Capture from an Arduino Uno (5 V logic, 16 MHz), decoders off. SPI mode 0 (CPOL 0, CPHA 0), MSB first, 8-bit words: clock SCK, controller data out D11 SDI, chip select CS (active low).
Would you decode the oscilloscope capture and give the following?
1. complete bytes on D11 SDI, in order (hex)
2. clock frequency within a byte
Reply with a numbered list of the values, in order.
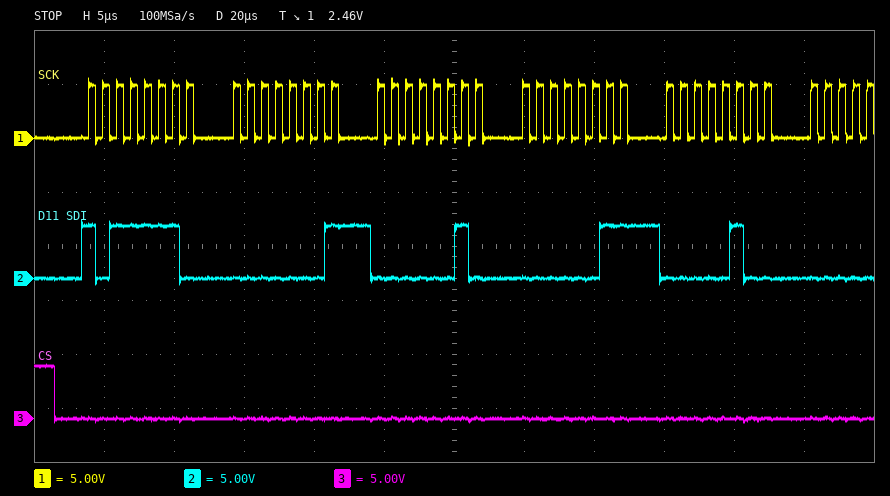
1. BE 01 02 03 04
2. 1 MHz
